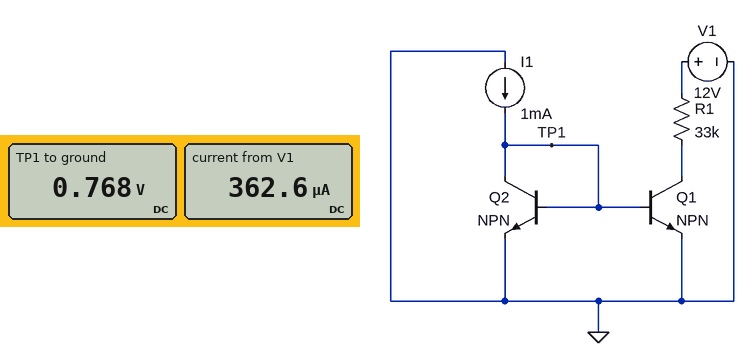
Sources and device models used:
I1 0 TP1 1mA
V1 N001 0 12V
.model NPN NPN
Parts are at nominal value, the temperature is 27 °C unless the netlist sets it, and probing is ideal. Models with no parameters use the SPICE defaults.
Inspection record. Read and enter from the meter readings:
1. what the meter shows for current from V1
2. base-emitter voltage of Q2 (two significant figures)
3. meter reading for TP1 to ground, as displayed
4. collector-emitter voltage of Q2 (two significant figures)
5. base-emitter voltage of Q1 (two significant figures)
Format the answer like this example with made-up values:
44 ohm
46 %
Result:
362.6 µA
770 mV
0.768 V
770 mV
770 mV
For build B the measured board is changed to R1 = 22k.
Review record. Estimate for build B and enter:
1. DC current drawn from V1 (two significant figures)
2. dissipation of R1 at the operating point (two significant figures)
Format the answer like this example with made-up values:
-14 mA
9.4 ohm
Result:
540 µA
6.5 mW
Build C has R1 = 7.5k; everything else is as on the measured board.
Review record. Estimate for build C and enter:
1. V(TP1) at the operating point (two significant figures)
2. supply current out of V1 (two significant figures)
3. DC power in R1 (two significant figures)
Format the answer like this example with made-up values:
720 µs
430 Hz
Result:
770 mV
980 µA
7.2 mW
